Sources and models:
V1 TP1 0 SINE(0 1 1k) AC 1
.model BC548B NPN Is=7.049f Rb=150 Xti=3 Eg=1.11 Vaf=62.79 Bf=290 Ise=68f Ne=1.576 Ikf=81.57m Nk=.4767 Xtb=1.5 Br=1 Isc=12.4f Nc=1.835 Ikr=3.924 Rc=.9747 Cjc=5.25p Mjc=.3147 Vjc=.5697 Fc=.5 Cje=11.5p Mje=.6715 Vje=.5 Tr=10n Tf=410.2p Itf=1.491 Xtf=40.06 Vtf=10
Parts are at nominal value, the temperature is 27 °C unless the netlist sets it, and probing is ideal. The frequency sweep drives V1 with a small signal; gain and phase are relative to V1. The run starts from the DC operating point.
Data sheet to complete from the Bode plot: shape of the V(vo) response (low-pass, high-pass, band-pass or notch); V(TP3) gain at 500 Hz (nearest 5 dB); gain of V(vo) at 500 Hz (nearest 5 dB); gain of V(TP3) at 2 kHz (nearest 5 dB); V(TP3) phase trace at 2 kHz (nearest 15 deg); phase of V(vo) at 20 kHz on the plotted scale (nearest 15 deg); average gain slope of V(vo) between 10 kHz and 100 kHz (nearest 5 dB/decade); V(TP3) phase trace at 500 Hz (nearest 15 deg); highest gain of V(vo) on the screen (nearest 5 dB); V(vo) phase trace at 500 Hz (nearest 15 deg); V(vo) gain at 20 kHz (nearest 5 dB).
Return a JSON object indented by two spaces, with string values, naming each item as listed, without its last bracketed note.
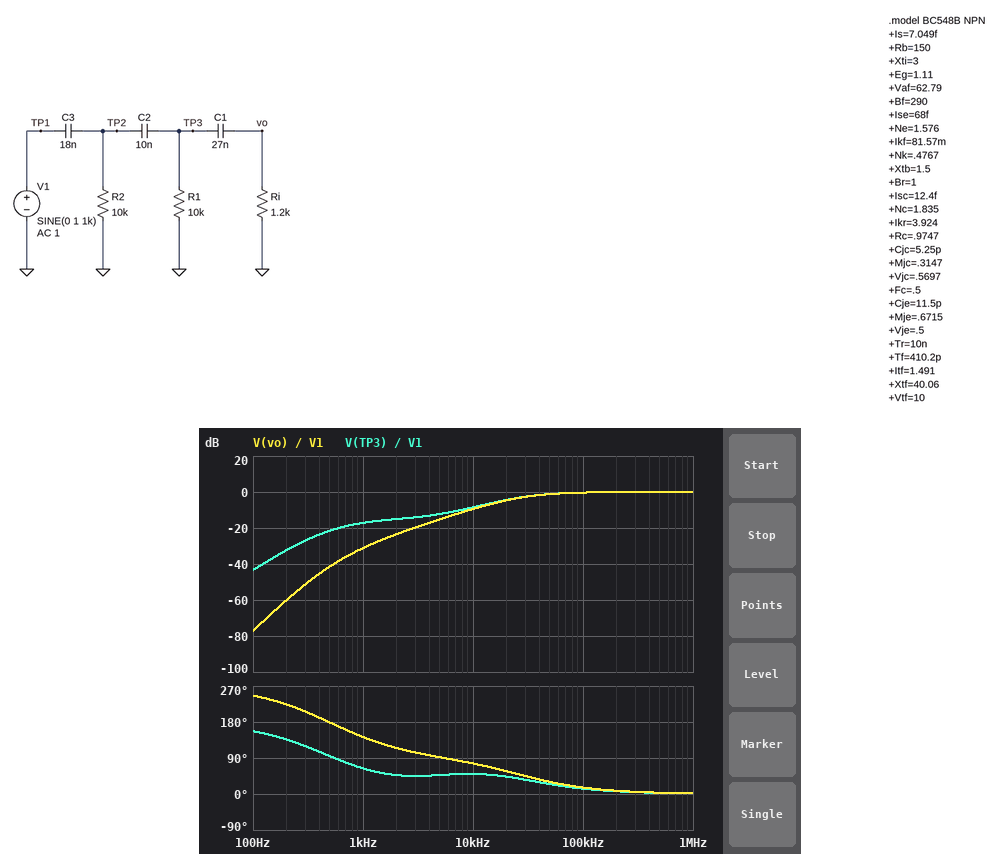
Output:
{
  "shape of the V(vo) response": "high-pass",
  "V(TP3) gain at 500 Hz": "-20 dB",
  "gain of V(vo) at 500 Hz": "-40 dB",
  "gain of V(TP3) at 2 kHz": "-15 dB",
  "V(TP3) phase trace at 2 kHz": "45 deg",
  "phase of V(vo) at 20 kHz on the plotted scale": "60 deg",
  "average gain slope of V(vo) between 10 kHz and 100 kHz": "10 dB/decade",
  "V(TP3) phase trace at 500 Hz": "90 deg",
  "highest gain of V(vo) on the screen": "0 dB",
  "V(vo) phase trace at 500 Hz": "180 deg",
  "V(vo) gain at 20 kHz": "-5 dB"
}
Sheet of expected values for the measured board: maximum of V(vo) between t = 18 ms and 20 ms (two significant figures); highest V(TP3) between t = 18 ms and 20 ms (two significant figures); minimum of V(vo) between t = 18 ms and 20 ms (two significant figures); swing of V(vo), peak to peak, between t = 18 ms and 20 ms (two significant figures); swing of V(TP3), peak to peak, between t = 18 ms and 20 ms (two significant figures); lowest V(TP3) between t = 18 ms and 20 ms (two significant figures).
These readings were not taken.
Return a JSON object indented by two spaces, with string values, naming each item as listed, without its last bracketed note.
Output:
{
  "maximum of V(vo) between t = 18 ms and 20 ms": "28 mV",
  "highest V(TP3) between t = 18 ms and 20 ms": "140 mV",
  "minimum of V(vo) between t = 18 ms and 20 ms": "-28 mV",
  "swing of V(vo), peak to peak, between t = 18 ms and 20 ms": "55 mV",
  "swing of V(TP3), peak to peak, between t = 18 ms and 20 ms": "280 mV",
  "lowest V(TP3) between t = 18 ms and 20 ms": "-140 mV"
}
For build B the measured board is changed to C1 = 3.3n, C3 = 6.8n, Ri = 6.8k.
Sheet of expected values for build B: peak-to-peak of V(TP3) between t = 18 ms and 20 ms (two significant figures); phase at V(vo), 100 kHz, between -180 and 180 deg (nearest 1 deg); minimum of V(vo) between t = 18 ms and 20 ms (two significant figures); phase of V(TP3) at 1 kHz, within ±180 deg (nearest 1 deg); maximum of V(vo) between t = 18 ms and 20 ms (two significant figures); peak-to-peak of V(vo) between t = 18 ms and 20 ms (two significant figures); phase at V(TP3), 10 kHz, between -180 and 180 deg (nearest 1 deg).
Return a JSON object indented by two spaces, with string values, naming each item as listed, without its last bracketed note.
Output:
{
  "peak-to-peak of V(TP3) between t = 18 ms and 20 ms": "270 mV",
  "phase at V(vo), 100 kHz, between -180 and 180 deg": "11 deg",
  "minimum of V(vo) between t = 18 ms and 20 ms": "-19 mV",
  "phase of V(TP3) at 1 kHz, within ±180 deg": "106 deg",
  "maximum of V(vo) between t = 18 ms and 20 ms": "19 mV",
  "peak-to-peak of V(vo) between t = 18 ms and 20 ms": "38 mV",
  "phase at V(TP3), 10 kHz, between -180 and 180 deg": "41 deg"
}
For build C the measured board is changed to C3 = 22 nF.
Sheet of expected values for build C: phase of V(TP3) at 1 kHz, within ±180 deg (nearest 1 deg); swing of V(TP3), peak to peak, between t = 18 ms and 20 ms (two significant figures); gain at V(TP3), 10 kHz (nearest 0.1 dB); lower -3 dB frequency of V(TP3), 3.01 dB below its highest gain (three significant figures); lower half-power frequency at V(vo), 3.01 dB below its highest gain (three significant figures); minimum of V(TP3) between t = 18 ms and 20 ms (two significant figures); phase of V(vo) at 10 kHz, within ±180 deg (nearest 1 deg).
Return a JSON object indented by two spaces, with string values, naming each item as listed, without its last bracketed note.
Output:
{
  "phase of V(TP3) at 1 kHz, within ±180 deg": "60 deg",
  "swing of V(TP3), peak to peak, between t = 18 ms and 20 ms": "310 mV",
  "gain at V(TP3), 10 kHz": "-8.1 dB",
  "lower -3 dB frequency of V(TP3), 3.01 dB below its highest gain": "25.4 kHz",
  "lower half-power frequency at V(vo), 3.01 dB below its highest gain": "26.3 kHz",
  "minimum of V(TP3) between t = 18 ms and 20 ms": "-150 mV",
  "phase of V(vo) at 10 kHz, within ±180 deg": "75 deg"
}
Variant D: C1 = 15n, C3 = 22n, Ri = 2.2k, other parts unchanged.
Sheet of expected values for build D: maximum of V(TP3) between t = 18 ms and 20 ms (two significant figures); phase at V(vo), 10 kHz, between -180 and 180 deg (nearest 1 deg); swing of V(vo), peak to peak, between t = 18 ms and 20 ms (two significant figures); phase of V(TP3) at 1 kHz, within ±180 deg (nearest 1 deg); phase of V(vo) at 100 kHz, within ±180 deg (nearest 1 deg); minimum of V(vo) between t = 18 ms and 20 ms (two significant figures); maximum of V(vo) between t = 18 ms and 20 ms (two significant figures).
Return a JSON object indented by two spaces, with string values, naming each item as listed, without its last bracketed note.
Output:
{
  "maximum of V(TP3) between t = 18 ms and 20 ms": "210 mV",
  "phase at V(vo), 10 kHz, between -180 and 180 deg": "67 deg",
  "swing of V(vo), peak to peak, between t = 18 ms and 20 ms": "84 mV",
  "phase of V(TP3) at 1 kHz, within ±180 deg": "69 deg",
  "phase of V(vo) at 100 kHz, within ±180 deg": "10 deg",
  "minimum of V(vo) between t = 18 ms and 20 ms": "-42 mV",
  "maximum of V(vo) between t = 18 ms and 20 ms": "42 mV"
}
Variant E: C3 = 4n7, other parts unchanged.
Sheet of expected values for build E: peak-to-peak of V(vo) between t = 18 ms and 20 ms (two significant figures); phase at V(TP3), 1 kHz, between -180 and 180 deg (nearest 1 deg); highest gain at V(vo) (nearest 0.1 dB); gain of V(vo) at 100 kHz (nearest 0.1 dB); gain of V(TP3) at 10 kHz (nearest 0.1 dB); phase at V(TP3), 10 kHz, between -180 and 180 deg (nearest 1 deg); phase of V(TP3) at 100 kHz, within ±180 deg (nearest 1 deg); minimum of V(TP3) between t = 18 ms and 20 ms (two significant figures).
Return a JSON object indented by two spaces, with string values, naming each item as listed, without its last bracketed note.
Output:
{
  "peak-to-peak of V(vo) between t = 18 ms and 20 ms": "21 mV",
  "phase at V(TP3), 1 kHz, between -180 and 180 deg": "84 deg",
  "highest gain at V(vo)": "0 dB",
  "gain of V(vo) at 100 kHz": "-1.1 dB",
  "gain of V(TP3) at 10 kHz": "-13.8 dB",
  "phase at V(TP3), 10 kHz, between -180 and 180 deg": "63 deg",
  "phase of V(TP3) at 100 kHz, within ±180 deg": "26 deg",
  "minimum of V(TP3) between t = 18 ms and 20 ms": "-53 mV"
}
